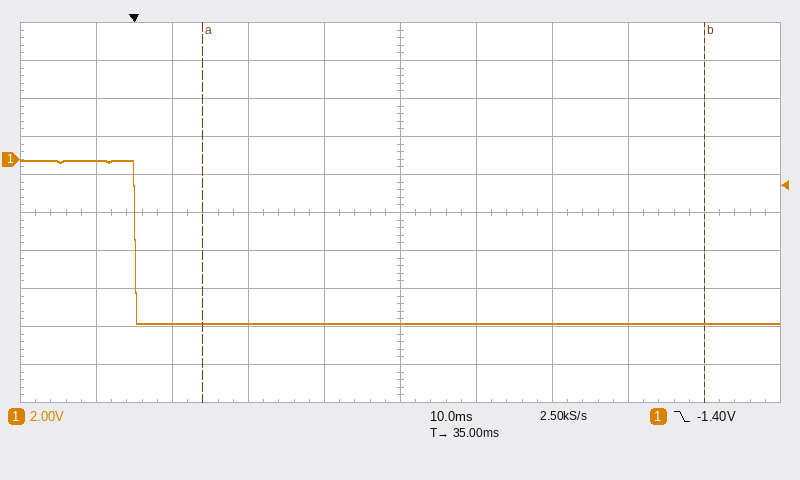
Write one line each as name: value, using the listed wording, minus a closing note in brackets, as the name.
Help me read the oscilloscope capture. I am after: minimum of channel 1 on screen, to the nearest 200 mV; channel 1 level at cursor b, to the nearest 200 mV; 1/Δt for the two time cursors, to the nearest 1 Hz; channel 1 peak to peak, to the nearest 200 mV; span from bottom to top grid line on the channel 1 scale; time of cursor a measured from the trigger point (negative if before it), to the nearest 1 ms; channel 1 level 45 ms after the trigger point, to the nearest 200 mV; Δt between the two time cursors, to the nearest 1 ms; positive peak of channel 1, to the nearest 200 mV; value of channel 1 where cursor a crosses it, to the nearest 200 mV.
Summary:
minimum of channel 1 on screen, to the nearest 200 mV: -8.6 V
channel 1 level at cursor b, to the nearest 200 mV: -8.6 V
1/Δt for the two time cursors, to the nearest 1 Hz: 15 Hz
channel 1 peak to peak, to the nearest 200 mV: 8.6 V
span from bottom to top grid line on the channel 1 scale: 20 V
time of cursor a measured from the trigger point (negative if before it), to the nearest 1 ms: +9 ms
channel 1 level 45 ms after the trigger point, to the nearest 200 mV: -8.6 V
Δt between the two time cursors, to the nearest 1 ms: 66 ms
positive peak of channel 1, to the nearest 200 mV: 0.0 V
value of channel 1 where cursor a crosses it, to the nearest 200 mV: -8.6 V
